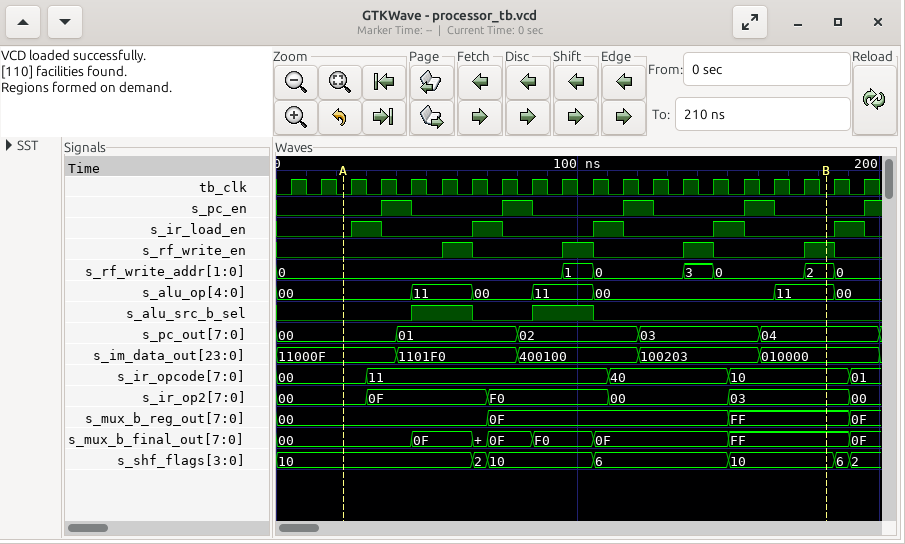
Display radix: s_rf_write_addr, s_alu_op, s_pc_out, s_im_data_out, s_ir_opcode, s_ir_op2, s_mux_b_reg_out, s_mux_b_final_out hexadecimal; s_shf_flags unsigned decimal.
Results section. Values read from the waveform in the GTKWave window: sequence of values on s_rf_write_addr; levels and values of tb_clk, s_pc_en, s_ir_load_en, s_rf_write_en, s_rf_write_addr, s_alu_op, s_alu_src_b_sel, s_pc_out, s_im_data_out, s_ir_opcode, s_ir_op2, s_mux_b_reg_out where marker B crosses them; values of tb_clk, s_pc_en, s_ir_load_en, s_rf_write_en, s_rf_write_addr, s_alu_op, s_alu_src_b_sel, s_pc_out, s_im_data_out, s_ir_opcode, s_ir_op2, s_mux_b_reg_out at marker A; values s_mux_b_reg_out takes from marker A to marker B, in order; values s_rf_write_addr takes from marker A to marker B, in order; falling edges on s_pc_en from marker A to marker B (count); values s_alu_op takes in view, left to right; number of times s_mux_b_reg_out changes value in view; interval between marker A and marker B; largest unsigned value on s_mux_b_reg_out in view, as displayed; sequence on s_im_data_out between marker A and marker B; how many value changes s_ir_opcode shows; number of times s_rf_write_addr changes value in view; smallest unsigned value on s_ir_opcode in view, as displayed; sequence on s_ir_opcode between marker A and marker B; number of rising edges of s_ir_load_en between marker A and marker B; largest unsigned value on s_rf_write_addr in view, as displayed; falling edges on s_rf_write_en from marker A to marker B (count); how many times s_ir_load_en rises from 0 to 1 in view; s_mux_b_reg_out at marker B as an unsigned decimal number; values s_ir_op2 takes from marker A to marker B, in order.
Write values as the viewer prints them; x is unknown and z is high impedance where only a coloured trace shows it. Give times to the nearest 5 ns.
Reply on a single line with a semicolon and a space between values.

0, 1, 0, 3, 0, 2, 0; tb_clk=0, s_pc_en=0, s_ir_load_en=0, s_rf_write_en=1, s_rf_write_addr=2, s_alu_op=11, s_alu_src_b_sel=0, s_pc_out=04, s_im_data_out=010000, s_ir_opcode=10, s_ir_op2=03, s_mux_b_reg_out=FF; tb_clk=0, s_pc_en=0, s_ir_load_en=0, s_rf_write_en=0, s_rf_write_addr=0, s_alu_op=00, s_alu_src_b_sel=0, s_pc_out=00, s_im_data_out=11000F, s_ir_opcode=00, s_ir_op2=00, s_mux_b_reg_out=00; 00, 0F, FF; 0, 1, 0, 3, 0, 2; 4; 00, 11, 00, 11, 00, 11, 00; 3; 160 ns; FF; 11000F, 1101F0, 400100, 100203, 010000; 4; 6; 00; 00, 11, 40, 10; 4; 3; 3; 5; 255; 00, 0F, F0, 00, 03
